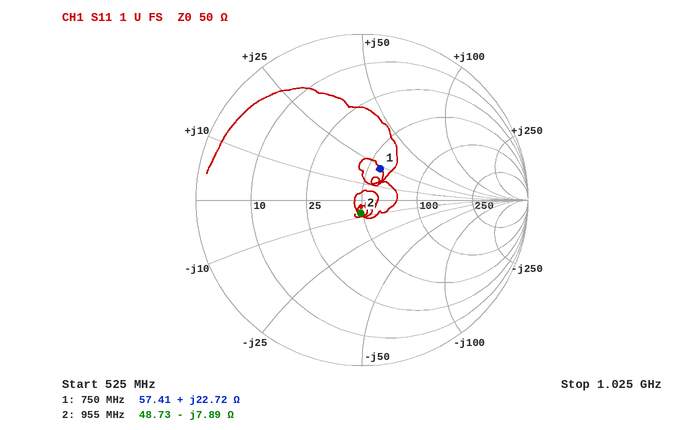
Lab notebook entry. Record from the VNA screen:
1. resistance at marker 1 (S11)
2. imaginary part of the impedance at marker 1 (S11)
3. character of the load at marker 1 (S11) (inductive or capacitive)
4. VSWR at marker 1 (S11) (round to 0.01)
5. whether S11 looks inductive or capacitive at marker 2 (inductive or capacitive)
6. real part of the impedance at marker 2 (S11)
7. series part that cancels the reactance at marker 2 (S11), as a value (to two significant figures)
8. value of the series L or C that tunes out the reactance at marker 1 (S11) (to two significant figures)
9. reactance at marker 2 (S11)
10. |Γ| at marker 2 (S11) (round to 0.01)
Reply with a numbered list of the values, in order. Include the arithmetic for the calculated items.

1. 57.41 Ω
2. +22.72 Ω
3. inductive
4. 1.56
5. capacitive
6. 48.73 Ω
7. L = 7.89 Ω/(2π × 955 MHz) ≈ 1.3 nH
8. C = 1/(2π × 750 MHz × 22.72 Ω) ≈ 9.3 pF
9. -7.89 Ω
10. 0.08
